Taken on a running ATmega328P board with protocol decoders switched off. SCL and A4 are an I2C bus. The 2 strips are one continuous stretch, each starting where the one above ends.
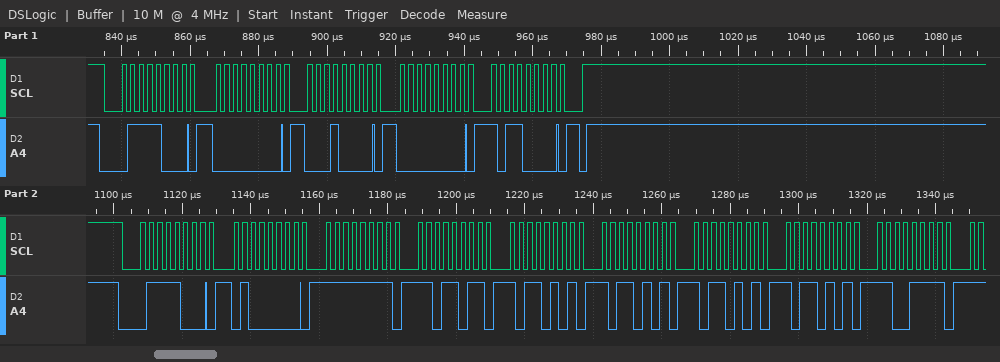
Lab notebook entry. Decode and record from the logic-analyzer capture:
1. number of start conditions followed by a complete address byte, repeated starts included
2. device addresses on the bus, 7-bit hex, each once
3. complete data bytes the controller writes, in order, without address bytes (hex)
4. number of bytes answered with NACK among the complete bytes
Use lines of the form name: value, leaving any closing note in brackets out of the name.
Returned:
number of start conditions followed by a complete address byte, repeated starts included: 2
device addresses on the bus, 7-bit hex, each once: 0x3C
complete data bytes the controller writes, in order, without address bytes: 00 10 00 B0 40 FF DB B5 B5 B5 B5 CF
number of bytes answered with NACK among the complete bytes: 0
